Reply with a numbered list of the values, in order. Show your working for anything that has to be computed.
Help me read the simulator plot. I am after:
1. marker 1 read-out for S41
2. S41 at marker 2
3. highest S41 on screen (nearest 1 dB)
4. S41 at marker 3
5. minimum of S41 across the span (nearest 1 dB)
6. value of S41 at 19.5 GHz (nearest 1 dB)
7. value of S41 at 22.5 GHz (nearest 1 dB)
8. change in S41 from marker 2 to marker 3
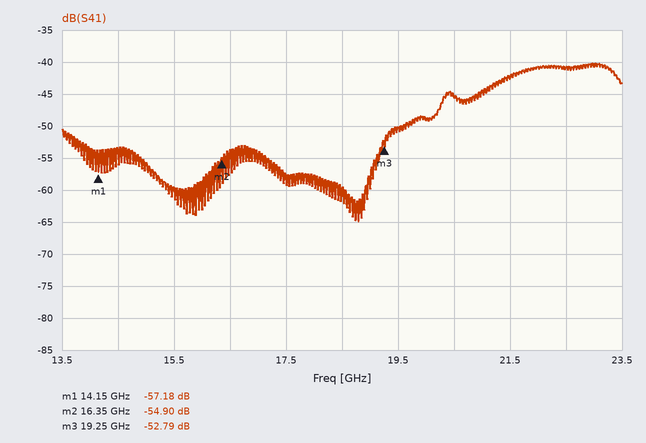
1. -57.18 dB
2. -54.90 dB
3. -40 dB
4. -52.79 dB
5. -65 dB
6. -50 dB
7. -41 dB
8. -52.79 − (-54.9) = 2.11 dB
